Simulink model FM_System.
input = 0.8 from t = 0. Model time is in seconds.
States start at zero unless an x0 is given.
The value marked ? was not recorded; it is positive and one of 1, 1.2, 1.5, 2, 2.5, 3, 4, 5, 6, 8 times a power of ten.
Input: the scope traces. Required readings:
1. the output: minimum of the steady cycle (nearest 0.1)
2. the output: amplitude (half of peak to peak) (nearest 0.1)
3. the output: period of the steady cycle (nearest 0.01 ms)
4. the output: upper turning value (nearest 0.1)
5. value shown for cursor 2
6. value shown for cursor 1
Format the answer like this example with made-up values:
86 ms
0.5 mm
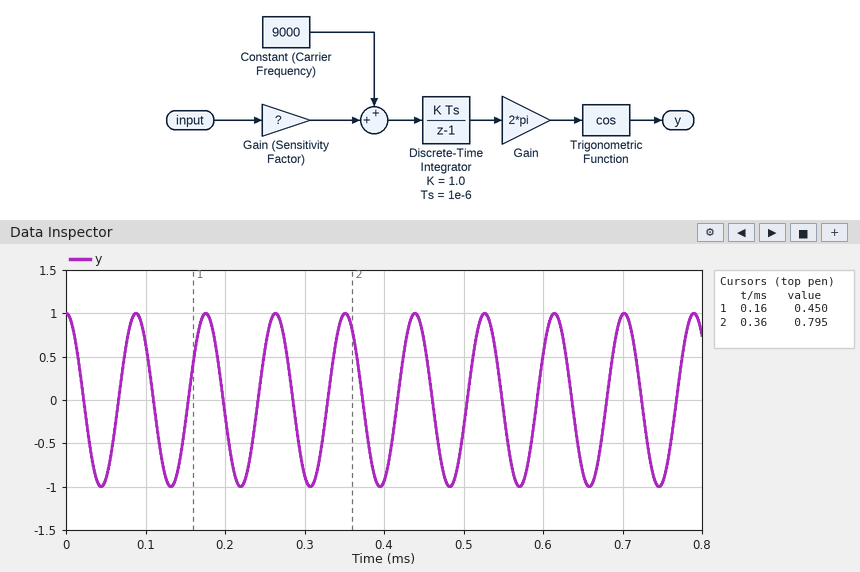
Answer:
-1.0
1.0
0.09 ms
1.0
0.795
0.450
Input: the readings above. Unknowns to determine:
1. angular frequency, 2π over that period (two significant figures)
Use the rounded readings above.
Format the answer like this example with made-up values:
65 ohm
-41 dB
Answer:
70 rad/ms
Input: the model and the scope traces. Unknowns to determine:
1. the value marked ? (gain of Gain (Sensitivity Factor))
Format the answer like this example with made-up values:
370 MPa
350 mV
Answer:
3000
